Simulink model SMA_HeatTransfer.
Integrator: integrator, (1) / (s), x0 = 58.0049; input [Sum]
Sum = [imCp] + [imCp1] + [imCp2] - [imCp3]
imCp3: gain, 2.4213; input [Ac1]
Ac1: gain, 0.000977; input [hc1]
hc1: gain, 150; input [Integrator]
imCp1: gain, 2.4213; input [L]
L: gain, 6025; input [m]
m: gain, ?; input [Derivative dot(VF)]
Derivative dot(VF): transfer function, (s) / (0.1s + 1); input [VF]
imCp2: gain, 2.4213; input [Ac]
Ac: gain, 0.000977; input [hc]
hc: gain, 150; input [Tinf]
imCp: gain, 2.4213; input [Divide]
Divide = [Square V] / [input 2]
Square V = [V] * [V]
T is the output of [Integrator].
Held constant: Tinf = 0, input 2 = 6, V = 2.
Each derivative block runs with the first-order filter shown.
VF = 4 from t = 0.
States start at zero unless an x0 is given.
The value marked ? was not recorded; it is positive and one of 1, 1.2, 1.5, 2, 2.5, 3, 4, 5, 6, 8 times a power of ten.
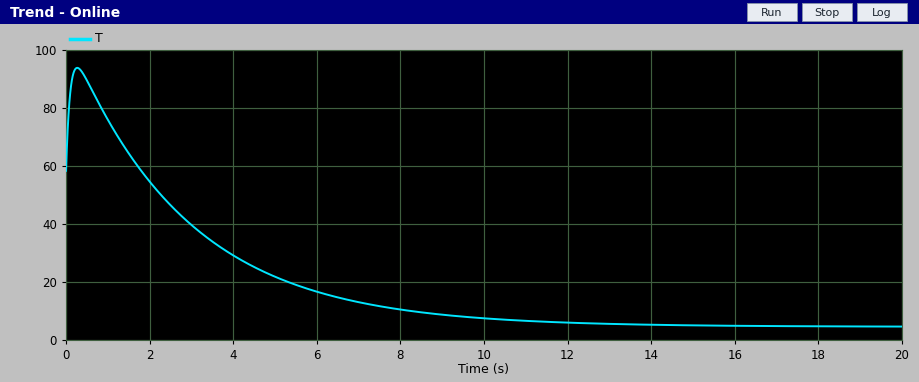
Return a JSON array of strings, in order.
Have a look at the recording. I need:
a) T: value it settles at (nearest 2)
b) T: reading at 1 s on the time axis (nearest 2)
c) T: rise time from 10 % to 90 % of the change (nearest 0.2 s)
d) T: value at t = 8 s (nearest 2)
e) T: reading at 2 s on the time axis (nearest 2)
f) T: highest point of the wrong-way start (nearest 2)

["4", "76", "6.2 s", "10", "54", "94"]
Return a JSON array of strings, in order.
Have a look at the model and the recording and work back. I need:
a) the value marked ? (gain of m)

["0.0008"]
